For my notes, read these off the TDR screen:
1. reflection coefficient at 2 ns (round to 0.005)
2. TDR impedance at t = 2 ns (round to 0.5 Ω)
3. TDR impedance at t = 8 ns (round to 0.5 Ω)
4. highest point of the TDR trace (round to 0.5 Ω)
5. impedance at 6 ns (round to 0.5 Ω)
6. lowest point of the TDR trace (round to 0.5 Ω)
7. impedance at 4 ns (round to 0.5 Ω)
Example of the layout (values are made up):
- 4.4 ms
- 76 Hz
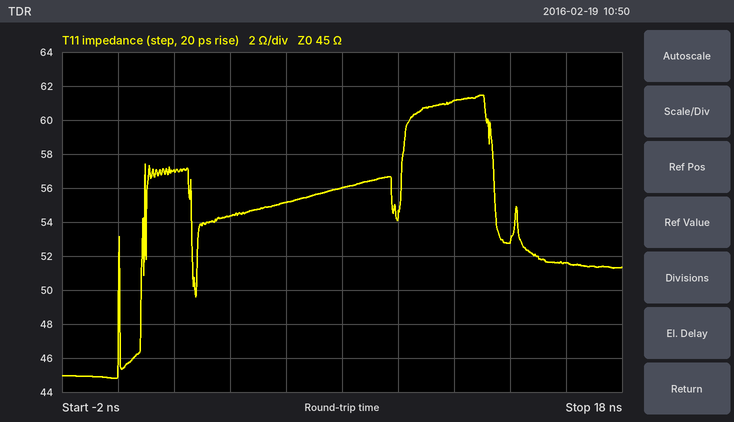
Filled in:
- +0.120
- 57.0 Ω
- 56.0 Ω
- 61.5 Ω
- 55.0 Ω
- 45.0 Ω
- 54.5 Ω
